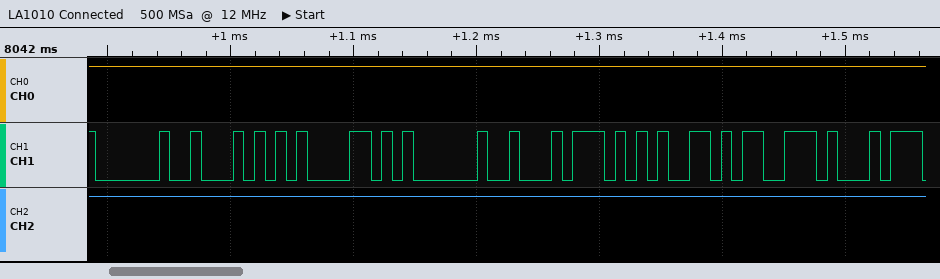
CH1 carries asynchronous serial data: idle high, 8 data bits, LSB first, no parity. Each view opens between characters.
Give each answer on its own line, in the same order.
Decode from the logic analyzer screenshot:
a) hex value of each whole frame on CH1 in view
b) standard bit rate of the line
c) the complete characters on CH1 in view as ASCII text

20, 54, 58, 20, 74, 65, 73
115200 baud
" TX tes"
